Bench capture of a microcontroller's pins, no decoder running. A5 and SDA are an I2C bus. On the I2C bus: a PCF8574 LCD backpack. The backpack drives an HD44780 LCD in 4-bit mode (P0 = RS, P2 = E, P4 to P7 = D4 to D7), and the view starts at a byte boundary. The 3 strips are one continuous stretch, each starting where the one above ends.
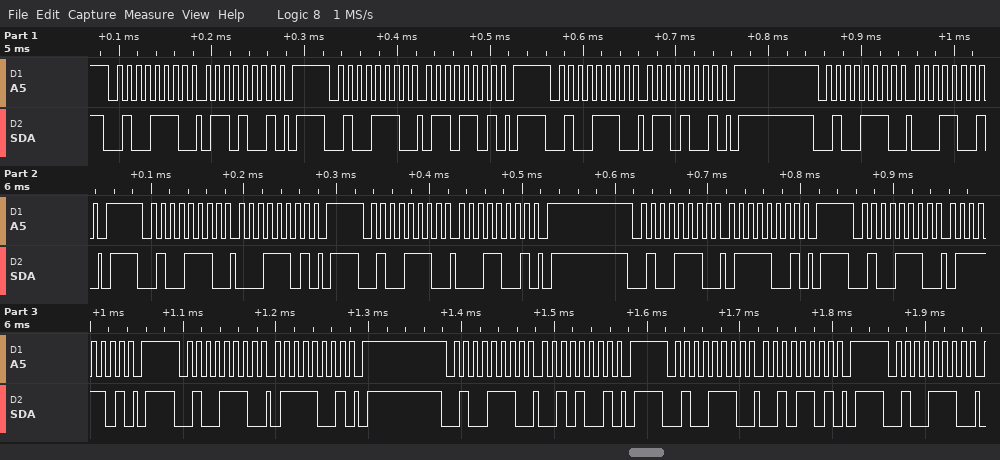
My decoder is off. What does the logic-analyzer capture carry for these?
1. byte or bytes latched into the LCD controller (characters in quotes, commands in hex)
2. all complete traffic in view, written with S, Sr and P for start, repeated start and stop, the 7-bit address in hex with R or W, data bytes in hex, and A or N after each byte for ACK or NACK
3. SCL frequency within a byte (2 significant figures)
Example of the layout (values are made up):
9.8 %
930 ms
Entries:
'a'
S 27W A 69 A P S 27W A 6D A P S 27W A 69 A P S 27W A 19 A P S 27W A 1D A P S 27W A 19 A P S 27W A 79 A P S 27W A 7D A P S 27W A 79 A P S 27W A 29 A P S 27W A 2D A P S 27W A
100 kHz
